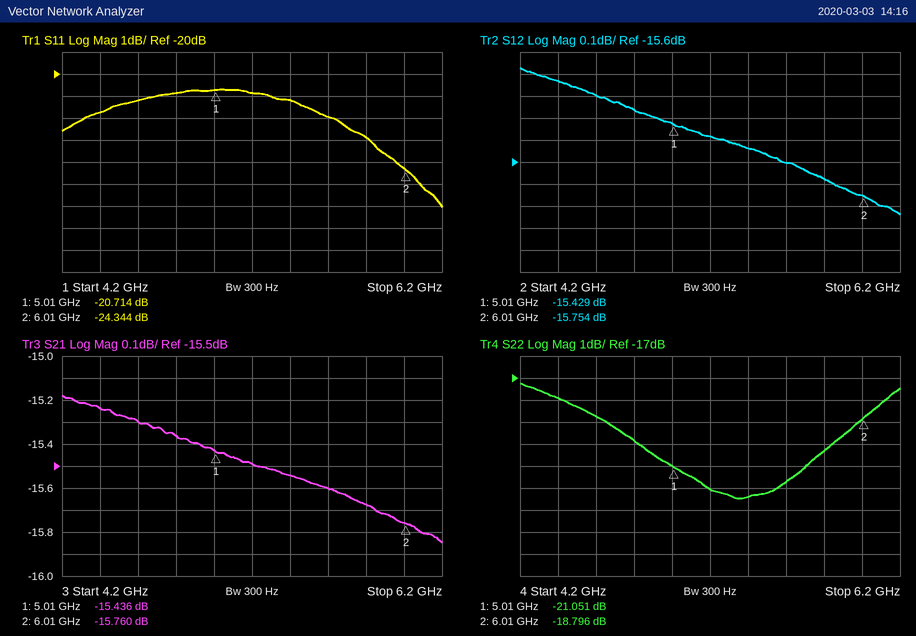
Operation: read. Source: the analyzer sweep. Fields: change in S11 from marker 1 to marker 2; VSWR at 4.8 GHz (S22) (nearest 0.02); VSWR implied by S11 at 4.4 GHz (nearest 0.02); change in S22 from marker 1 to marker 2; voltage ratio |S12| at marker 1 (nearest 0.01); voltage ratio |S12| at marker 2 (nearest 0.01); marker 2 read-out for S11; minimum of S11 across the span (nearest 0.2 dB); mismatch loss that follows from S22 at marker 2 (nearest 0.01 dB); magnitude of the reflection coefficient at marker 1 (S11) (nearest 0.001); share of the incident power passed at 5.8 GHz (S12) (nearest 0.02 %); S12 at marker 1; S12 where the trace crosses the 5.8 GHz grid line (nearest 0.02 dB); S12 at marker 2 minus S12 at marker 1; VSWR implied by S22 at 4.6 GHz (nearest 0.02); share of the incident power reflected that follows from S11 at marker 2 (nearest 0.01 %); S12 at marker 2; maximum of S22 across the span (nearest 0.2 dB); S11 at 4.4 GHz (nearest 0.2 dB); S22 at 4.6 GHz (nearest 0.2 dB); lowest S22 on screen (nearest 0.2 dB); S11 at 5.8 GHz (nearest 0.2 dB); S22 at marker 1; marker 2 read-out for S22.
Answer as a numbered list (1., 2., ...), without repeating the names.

1. -3.630 dB
2. 1.22
3. 1.18
4. 2.255 dB
5. 0.17
6. 0.16
7. -24.344 dB
8. -26.0 dB
9. 0.06 dB
10. 0.092
11. 2.70 %
12. -15.429 dB
13. -15.68 dB
14. -0.325 dB
15. 1.26
16. 0.37 %
17. -15.754 dB
18. -17.2 dB
19. -21.8 dB
20. -18.8 dB
21. -22.4 dB
22. -22.8 dB
23. -21.051 dB
24. -18.796 dB
